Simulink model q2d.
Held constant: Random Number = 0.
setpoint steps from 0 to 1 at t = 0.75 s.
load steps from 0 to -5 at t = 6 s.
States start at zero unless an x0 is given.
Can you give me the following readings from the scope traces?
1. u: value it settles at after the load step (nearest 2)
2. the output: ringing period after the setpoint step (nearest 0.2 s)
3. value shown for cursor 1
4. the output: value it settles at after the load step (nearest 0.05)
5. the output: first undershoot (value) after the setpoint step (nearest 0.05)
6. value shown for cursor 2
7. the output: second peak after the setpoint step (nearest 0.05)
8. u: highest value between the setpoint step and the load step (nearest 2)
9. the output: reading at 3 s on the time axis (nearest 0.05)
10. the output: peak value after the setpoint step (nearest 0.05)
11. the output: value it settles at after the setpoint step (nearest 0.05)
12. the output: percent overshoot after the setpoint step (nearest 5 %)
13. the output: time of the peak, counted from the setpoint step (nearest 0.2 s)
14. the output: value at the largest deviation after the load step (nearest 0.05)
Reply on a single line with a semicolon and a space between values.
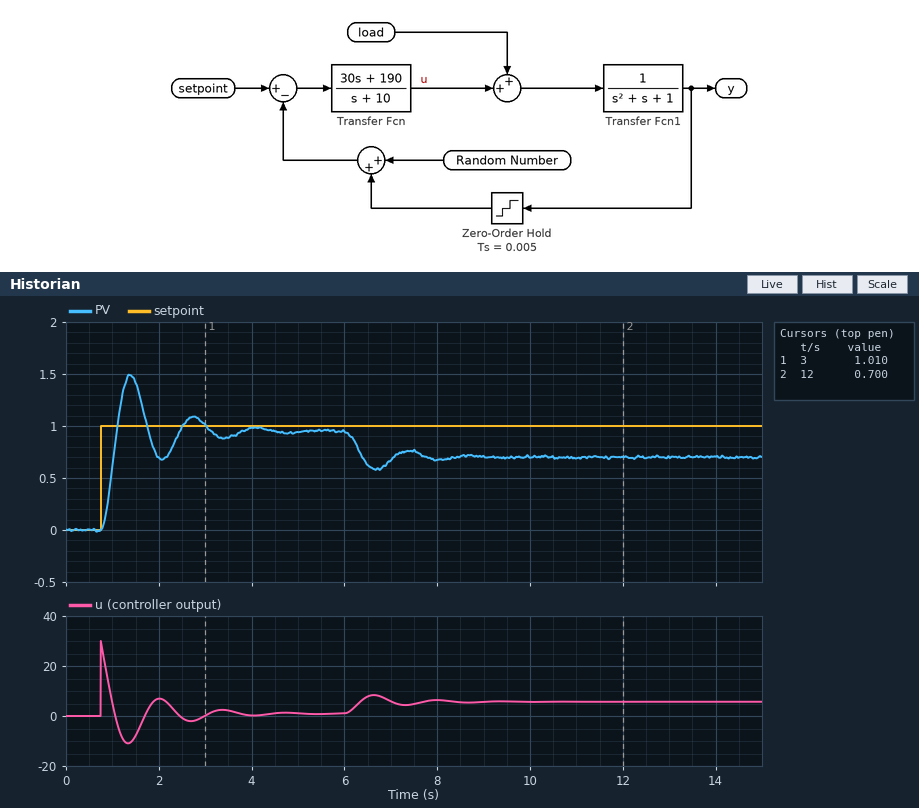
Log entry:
6; 1.4 s; 1.010; 0.70; 0.70; 0.700; 1.10; 30; 1.00; 1.50; 0.95; 55 %; 0.6 s; 0.60
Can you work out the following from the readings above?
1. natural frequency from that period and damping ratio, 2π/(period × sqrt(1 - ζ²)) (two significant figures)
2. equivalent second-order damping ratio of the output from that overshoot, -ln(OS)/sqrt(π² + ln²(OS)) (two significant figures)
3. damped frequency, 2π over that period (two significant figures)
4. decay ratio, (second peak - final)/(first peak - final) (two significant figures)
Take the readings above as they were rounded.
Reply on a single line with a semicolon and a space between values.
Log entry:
4.6 rad/s; 0.19; 4.5 rad/s; 0.27
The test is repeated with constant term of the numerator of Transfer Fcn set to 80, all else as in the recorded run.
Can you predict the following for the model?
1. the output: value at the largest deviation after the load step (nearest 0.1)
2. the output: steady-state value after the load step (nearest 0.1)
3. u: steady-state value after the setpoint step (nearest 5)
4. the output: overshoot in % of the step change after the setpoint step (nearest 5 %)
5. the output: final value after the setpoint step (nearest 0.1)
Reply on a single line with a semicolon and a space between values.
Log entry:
0.3; 0.3; 0; 30 %; 0.9
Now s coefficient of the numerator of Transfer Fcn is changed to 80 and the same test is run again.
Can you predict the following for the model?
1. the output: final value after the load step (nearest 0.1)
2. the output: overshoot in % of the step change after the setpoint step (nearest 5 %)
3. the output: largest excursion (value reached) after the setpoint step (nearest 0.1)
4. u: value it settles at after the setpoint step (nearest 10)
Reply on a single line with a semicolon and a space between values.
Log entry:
0.7; 35 %; 1.3; 0
